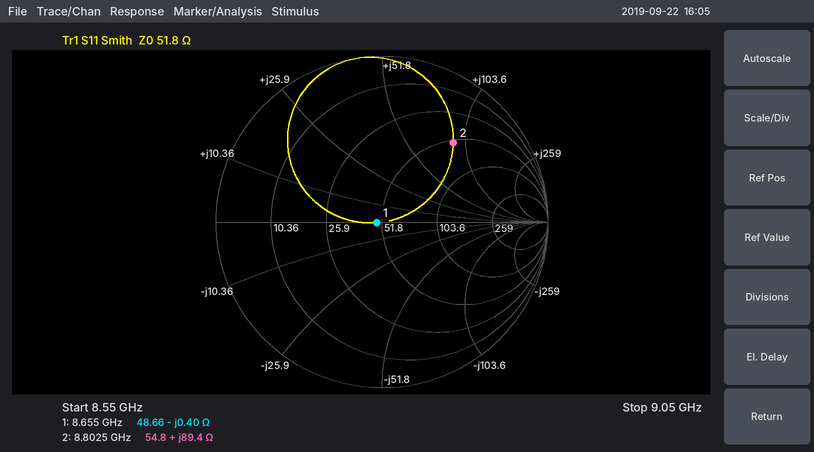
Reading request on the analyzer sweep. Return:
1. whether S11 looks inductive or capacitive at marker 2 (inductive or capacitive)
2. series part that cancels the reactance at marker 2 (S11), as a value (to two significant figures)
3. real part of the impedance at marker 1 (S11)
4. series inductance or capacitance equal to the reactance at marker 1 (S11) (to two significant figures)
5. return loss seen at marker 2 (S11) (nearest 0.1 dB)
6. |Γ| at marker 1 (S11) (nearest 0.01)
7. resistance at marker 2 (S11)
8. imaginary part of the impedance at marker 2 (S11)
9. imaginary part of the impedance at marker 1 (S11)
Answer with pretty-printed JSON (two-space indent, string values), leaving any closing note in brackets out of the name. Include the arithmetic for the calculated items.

{
  "whether S11 looks inductive or capacitive at marker 2": "inductive",
  "series part that cancels the reactance at marker 2 (S11), as a value": "C = 1/(2π × 8.8025 GHz × 89.4 Ω) ≈ 202 fF, so 200 fF to two significant figures",
  "real part of the impedance at marker 1": "48.66 Ω",
  "series inductance or capacitance equal to the reactance at marker 1 (S11)": "C = 1/(2π × 8.655 GHz × 0.4 Ω) ≈ 46 pF",
  "return loss seen at marker 2 (S11)": "3.8 dB",
  "|Γ| at marker 1 (S11)": "0.03",
  "resistance at marker 2": "54.8 Ω",
  "imaginary part of the impedance at marker 2": "+89.4 Ω",
  "imaginary part of the impedance at marker 1": "-0.40 Ω"
}
